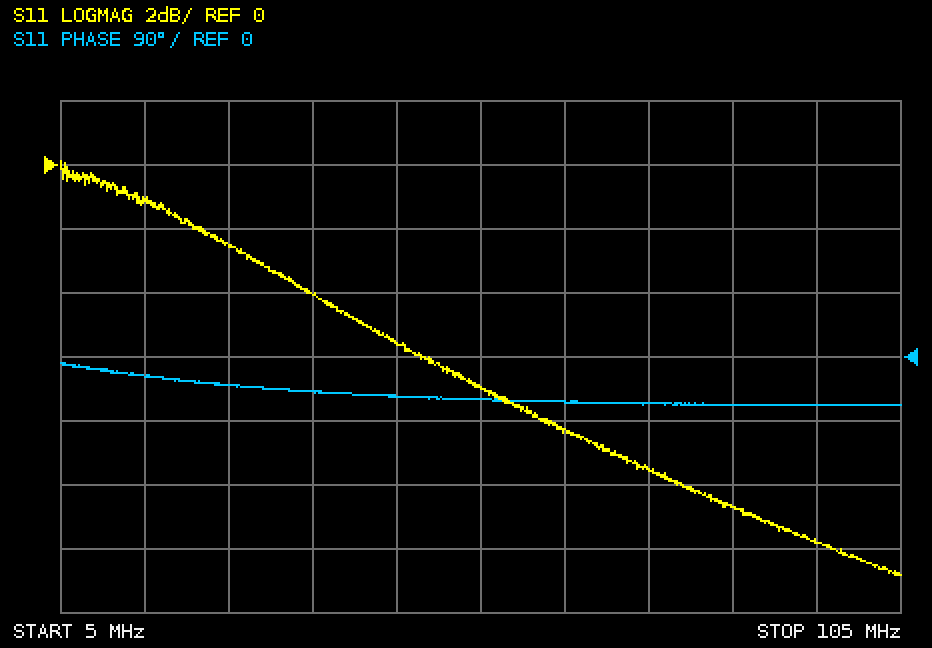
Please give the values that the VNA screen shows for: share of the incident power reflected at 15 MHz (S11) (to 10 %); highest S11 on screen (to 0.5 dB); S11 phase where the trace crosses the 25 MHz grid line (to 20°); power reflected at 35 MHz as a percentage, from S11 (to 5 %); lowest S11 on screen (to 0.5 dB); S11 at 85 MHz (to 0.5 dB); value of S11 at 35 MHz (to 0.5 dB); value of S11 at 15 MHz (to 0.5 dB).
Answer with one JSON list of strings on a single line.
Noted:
["80 %", "0.0 dB", "-40°", "40 %", "-13.0 dB", "-10.5 dB", "-4.0 dB", "-1.0 dB"]
